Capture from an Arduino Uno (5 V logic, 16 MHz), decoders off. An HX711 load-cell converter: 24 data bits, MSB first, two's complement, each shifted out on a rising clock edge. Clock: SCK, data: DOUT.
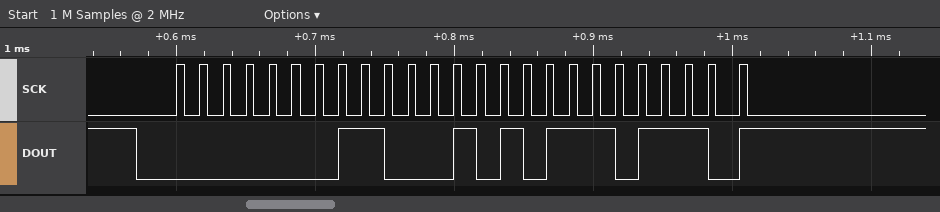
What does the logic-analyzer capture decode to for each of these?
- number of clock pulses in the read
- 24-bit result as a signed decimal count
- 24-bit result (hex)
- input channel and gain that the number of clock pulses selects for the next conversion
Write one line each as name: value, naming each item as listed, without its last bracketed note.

number of clock pulses in the read: 25
24-bit result as a signed decimal count: 101102
24-bit result: 0x018AEE
input channel and gain that the number of clock pulses selects for the next conversion: channel A, gain 128
